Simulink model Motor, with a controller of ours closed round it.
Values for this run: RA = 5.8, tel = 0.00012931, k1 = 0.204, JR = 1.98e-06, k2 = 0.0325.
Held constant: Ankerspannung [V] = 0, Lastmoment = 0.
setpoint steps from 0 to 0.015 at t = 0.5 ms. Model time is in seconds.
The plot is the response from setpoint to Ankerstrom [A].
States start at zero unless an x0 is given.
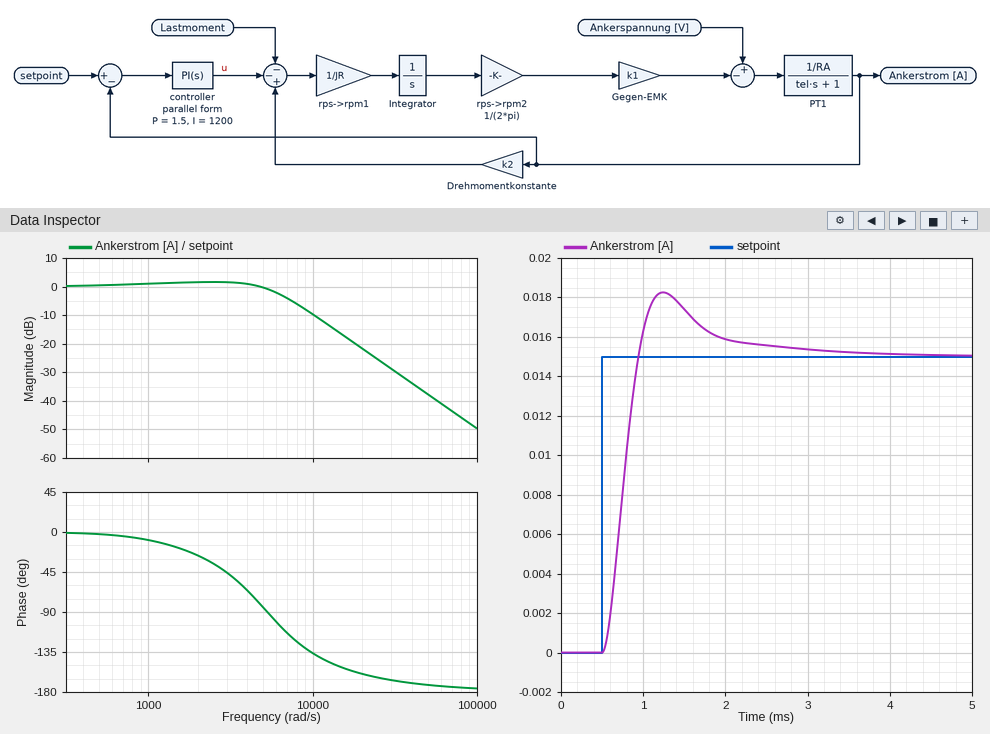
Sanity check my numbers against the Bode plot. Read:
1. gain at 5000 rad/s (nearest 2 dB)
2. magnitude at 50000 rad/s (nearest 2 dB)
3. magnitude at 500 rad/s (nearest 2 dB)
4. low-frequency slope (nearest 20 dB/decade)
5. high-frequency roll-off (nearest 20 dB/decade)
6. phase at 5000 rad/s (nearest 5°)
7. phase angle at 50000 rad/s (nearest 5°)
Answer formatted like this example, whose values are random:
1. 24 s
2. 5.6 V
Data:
1. 0 dB
2. -38 dB
3. 0 dB
4. 0 dB/decade
5. -40 dB/decade
6. -85°
7. -170°
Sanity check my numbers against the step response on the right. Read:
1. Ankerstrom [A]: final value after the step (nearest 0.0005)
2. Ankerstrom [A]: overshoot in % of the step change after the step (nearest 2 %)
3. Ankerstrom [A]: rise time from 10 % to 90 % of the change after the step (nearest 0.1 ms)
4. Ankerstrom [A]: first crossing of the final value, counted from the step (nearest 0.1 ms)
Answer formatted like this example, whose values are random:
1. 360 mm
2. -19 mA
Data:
1. 0.0150
2. 22 %
3. 0.3 ms
4. 0.4 ms
